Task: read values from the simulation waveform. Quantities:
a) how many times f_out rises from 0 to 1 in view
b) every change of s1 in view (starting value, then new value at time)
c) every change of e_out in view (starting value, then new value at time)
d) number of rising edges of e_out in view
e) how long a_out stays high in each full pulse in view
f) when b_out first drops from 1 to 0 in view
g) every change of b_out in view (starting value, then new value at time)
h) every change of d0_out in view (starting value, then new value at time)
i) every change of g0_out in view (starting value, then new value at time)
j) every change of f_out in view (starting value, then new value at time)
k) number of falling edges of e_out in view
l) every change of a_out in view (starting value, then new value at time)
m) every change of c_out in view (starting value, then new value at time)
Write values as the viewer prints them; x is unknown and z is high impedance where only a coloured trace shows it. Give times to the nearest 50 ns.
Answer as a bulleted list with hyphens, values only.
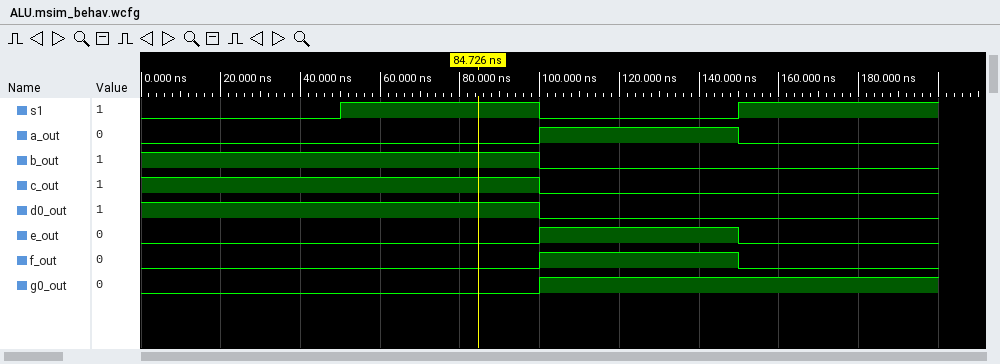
- 1
- 0, 1 at 50 ns, 0 at 100 ns, 1 at 150 ns
- 0, 1 at 100 ns, 0 at 150 ns
- 1
- 50 ns
- 100 ns
- 1, 0 at 100 ns
- 1, 0 at 100 ns
- 0, 1 at 100 ns
- 0, 1 at 100 ns, 0 at 150 ns
- 1
- 0, 1 at 100 ns, 0 at 150 ns
- 1, 0 at 100 ns
